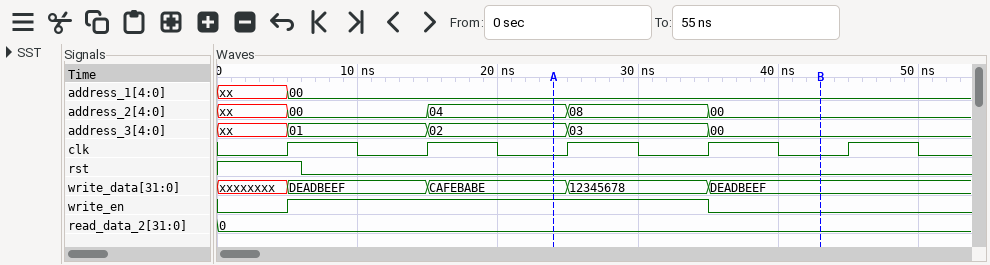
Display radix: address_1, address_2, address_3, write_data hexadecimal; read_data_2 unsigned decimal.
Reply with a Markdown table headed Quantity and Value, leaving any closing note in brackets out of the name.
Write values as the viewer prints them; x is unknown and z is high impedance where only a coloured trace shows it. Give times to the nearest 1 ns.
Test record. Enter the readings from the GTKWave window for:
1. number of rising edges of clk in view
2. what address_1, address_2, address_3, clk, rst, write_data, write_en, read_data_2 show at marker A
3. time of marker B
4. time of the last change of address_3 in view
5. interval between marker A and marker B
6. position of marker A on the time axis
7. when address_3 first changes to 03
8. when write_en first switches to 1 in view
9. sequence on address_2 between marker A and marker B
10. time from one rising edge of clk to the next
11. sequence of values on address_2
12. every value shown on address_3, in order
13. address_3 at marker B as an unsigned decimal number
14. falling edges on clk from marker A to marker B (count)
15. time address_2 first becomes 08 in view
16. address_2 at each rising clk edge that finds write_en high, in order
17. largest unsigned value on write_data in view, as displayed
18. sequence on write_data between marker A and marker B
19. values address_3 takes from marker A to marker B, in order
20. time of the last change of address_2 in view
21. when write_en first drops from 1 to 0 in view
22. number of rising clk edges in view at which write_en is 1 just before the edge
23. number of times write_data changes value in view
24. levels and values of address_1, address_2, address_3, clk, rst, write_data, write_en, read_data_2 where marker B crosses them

| Quantity | Value |
|---|---|
| number of rising edges of clk in view | 5 |
| what address_1, address_2, address_3, clk, rst, write_data, write_en, read_data_2 show at marker A | address_1=00, address_2=04, address_3=02, clk=0, rst=0, write_data=CAFEBABE, write_en=1, read_data_2=0 |
| time of marker B | 43 ns |
| time of the last change of address_3 in view | 35 ns |
| interval between marker A and marker B | 19 ns |
| position of marker A on the time axis | 24 ns |
| when address_3 first changes to 03 | 25 ns |
| when write_en first switches to 1 in view | 5 ns |
| sequence on address_2 between marker A and marker B | 04, 08, 00 |
| time from one rising edge of clk to the next | 10 ns |
| sequence of values on address_2 | xx, 00, 04, 08, 00 |
| every value shown on address_3, in order | xx, 01, 02, 03, 00 |
| address_3 at marker B as an unsigned decimal number | 0 |
| falling edges on clk from marker A to marker B | 2 |
| time address_2 first becomes 08 in view | 25 ns |
| address_2 at each rising clk edge that finds write_en high, in order | 00, 04, 08 |
| largest unsigned value on write_data in view, as displayed | DEADBEEF |
| sequence on write_data between marker A and marker B | CAFEBABE, 12345678, DEADBEEF |
| values address_3 takes from marker A to marker B, in order | 02, 03, 00 |
| time of the last change of address_2 in view | 35 ns |
| when write_en first drops from 1 to 0 in view | 35 ns |
| number of rising clk edges in view at which write_en is 1 just before the edge | 3 |
| number of times write_data changes value in view | 4 |
| levels and values of address_1, address_2, address_3, clk, rst, write_data, write_en, read_data_2 where marker B crosses them | address_1=00, address_2=00, address_3=00, clk=0, rst=0, write_data=DEADBEEF, write_en=0, read_data_2=0 |
